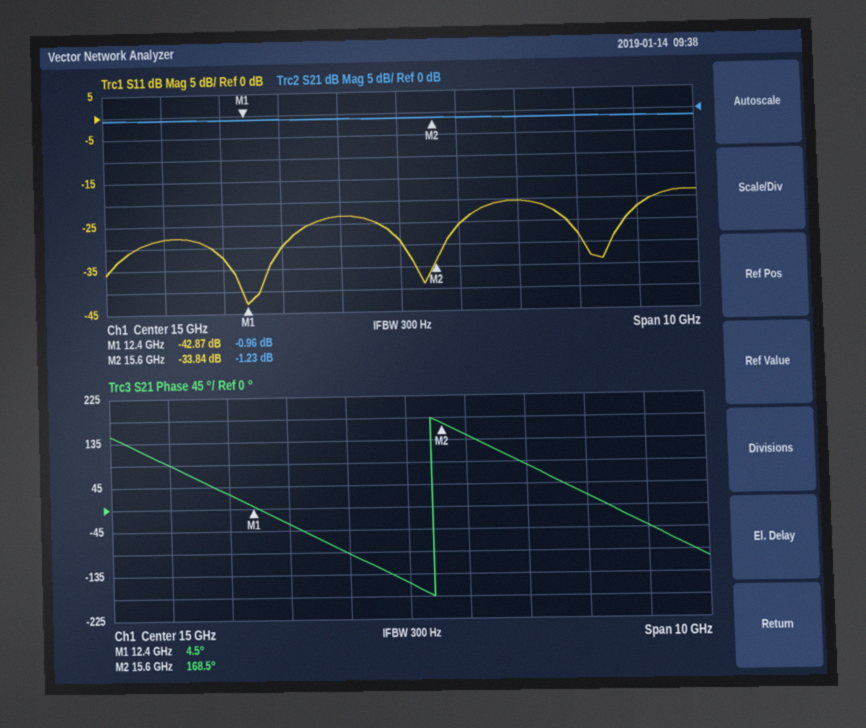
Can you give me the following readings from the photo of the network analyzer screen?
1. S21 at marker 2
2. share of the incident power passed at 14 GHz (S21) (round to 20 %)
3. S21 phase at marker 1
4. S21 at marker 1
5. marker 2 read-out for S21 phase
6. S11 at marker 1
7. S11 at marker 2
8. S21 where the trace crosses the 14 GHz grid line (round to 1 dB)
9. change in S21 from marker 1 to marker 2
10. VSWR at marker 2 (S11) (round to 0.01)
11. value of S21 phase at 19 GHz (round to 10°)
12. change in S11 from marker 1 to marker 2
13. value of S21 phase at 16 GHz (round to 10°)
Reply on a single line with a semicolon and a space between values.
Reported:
-1.23 dB; 80 %; 4.5°; -0.96 dB; 168.5°; -42.87 dB; -33.84 dB; -1 dB; -0.27 dB; 1.04; -40°; 9.03 dB; 140°
